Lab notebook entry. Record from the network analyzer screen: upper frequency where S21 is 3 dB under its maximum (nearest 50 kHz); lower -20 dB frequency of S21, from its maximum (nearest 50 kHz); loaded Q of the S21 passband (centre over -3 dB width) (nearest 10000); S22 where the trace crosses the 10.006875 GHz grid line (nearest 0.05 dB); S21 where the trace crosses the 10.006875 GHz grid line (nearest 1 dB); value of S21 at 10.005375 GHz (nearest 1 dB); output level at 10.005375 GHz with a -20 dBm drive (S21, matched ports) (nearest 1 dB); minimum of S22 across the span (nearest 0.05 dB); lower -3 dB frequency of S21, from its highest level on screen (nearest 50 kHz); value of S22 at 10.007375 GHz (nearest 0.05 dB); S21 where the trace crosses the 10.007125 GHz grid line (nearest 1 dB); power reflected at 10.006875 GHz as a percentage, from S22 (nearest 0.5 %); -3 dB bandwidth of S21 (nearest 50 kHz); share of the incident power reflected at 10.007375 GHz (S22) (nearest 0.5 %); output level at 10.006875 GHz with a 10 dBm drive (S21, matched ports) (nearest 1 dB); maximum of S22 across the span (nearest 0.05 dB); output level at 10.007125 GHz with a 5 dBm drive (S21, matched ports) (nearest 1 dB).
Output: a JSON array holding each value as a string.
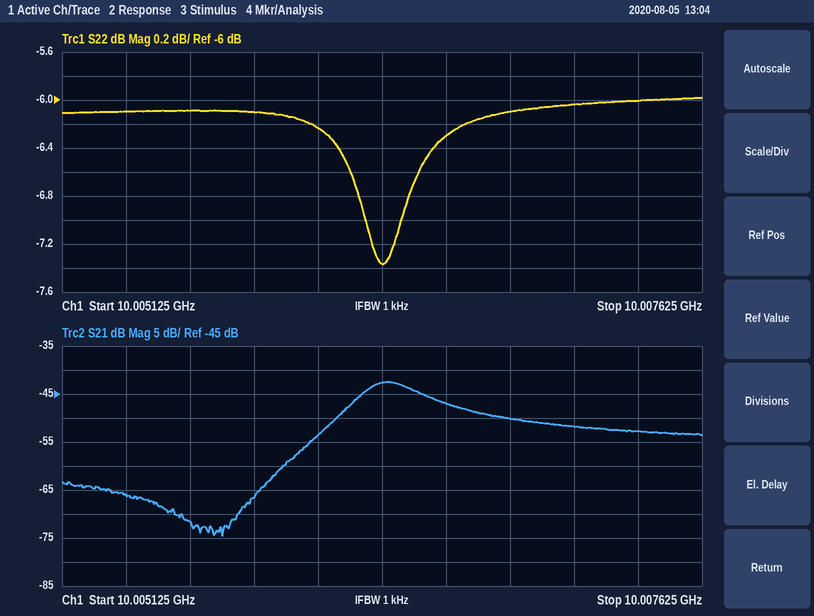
["10.00655 GHz", "10.00595 GHz", "40000", "-6.10 dB", "-50 dB", "-66 dB", "-86 dBm", "-7.35 dB", "10.00630 GHz", "-6.00 dB", "-52 dB", "24.5 %", "250 kHz", "25.0 %", "-40 dBm", "-6.00 dB", "-47 dBm"]
